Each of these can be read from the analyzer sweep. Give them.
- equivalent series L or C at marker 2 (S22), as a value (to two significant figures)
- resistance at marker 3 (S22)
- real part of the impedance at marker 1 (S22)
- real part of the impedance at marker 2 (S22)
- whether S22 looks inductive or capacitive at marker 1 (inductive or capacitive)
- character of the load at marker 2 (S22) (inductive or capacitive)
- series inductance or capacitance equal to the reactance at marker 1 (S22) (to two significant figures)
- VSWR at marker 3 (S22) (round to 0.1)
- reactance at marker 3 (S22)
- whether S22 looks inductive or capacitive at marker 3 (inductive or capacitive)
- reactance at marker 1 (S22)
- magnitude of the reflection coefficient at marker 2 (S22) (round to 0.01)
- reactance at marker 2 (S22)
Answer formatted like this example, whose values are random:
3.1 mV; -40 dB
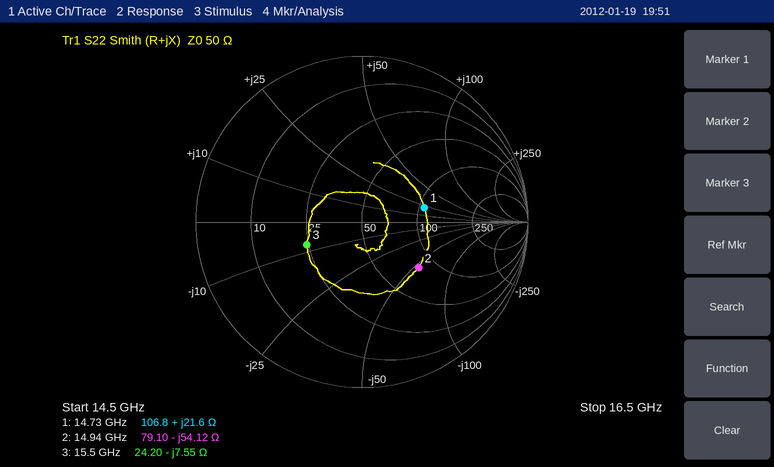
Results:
200 fF; 24.20 Ω; 106.8 Ω; 79.10 Ω; inductive; capacitive; 230 pH; 2.1; -7.55 Ω; capacitive; +21.6 Ω; 0.44; -54.12 Ω
